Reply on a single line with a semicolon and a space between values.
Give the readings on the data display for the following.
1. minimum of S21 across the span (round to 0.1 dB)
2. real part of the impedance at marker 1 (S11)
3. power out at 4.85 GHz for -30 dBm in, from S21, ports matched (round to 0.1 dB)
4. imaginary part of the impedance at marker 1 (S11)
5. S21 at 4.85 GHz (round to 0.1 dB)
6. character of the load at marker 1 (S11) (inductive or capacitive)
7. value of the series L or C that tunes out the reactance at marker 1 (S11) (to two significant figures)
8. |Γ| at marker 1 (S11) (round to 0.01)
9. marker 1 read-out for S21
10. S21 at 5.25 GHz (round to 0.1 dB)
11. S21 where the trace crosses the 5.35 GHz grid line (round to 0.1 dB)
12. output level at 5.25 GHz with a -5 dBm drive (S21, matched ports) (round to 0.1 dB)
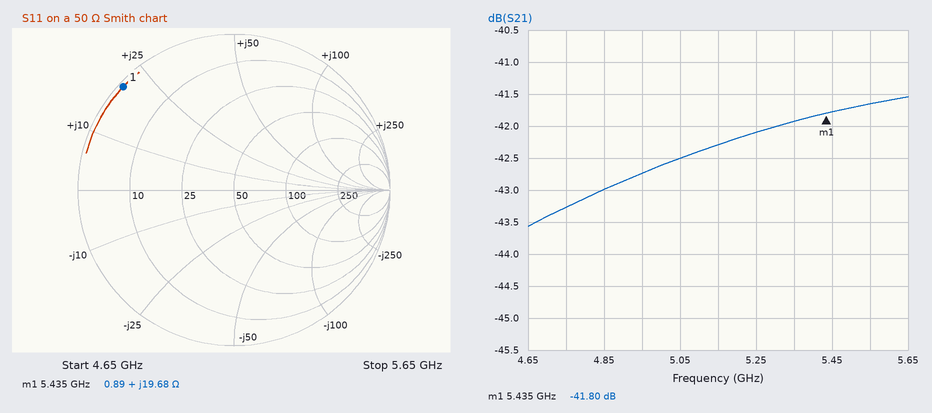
-43.6 dB; 0.89 Ω; -73.0 dBm; +19.68 Ω; -43.0 dB; inductive; 1.5 pF; 0.97; -41.80 dB; -42.1 dB; -41.9 dB; -47.1 dBm
